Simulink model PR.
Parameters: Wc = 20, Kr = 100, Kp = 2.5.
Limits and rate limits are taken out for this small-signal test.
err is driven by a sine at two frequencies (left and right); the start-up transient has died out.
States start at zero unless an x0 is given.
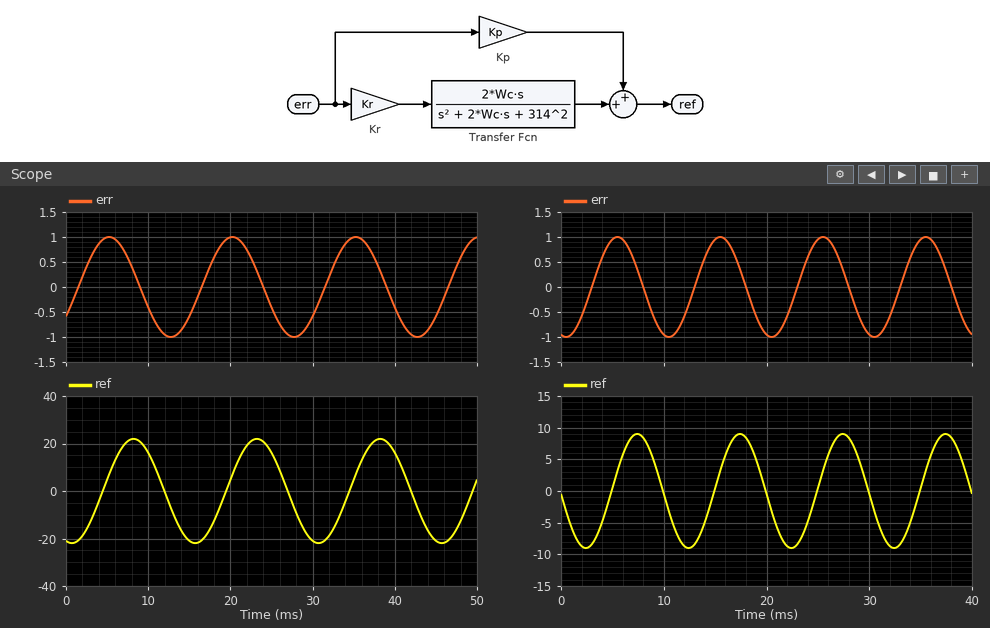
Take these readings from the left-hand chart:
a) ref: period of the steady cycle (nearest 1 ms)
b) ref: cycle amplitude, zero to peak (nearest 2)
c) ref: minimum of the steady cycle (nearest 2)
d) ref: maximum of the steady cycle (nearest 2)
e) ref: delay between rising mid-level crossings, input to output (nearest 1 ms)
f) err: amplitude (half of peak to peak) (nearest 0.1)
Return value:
15 ms
22
-22
22
3 ms
1.0
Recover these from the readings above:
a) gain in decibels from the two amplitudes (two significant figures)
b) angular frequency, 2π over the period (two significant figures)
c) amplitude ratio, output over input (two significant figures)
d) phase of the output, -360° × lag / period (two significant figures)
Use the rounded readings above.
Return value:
27 dB
0.42 rad/ms
22
-72°
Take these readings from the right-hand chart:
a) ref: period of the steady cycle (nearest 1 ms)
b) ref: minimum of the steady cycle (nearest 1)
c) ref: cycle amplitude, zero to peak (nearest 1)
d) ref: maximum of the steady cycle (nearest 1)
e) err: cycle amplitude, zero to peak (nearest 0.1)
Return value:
10 ms
-9
9
9
1.0
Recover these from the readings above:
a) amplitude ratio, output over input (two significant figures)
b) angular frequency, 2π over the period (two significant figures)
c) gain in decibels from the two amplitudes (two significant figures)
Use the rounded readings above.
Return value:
9.0
0.63 rad/ms
19 dB
